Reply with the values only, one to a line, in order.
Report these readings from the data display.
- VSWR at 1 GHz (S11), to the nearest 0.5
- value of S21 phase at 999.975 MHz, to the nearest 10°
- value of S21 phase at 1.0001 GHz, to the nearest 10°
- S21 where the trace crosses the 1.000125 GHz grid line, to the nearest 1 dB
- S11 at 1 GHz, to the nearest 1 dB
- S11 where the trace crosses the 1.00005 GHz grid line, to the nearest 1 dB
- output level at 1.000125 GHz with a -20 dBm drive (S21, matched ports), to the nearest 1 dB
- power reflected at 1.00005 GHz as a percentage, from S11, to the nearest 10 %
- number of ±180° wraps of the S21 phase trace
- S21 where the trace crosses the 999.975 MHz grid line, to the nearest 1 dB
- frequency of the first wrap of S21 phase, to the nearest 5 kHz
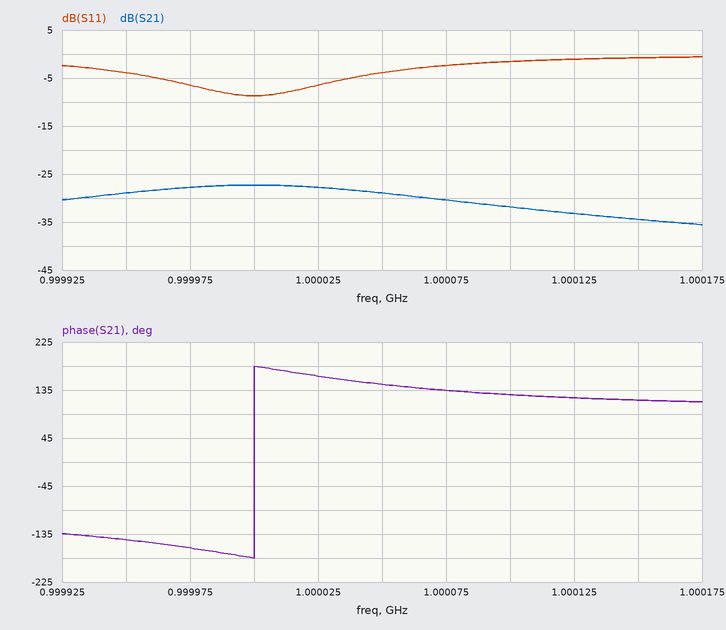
2.0
-160°
130°
-33 dB
-9 dB
-4 dB
-53 dBm
40 %
1
-28 dB
1.000000 GHz
